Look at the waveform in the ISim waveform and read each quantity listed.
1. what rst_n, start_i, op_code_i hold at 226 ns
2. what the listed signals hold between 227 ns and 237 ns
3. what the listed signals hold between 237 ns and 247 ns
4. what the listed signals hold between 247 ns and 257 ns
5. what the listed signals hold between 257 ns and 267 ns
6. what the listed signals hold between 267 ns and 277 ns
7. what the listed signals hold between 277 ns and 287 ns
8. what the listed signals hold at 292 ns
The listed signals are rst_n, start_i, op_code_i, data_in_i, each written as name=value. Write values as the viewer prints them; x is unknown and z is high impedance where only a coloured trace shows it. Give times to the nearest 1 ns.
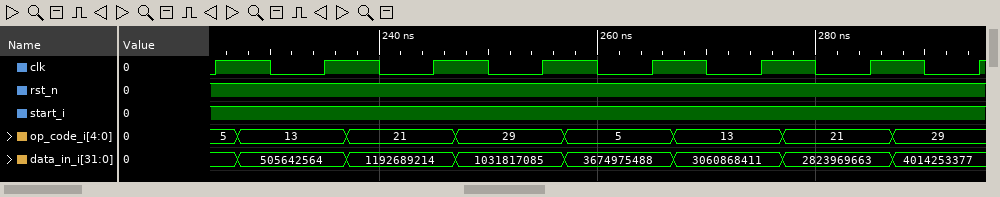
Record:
rst_n=1, start_i=1, op_code_i=5
rst_n=1, start_i=1, op_code_i=13, data_in_i=505642564
rst_n=1, start_i=1, op_code_i=21, data_in_i=1192689214
rst_n=1, start_i=1, op_code_i=29, data_in_i=1031817085
rst_n=1, start_i=1, op_code_i=5, data_in_i=3674975488
rst_n=1, start_i=1, op_code_i=13, data_in_i=3060868411
rst_n=1, start_i=1, op_code_i=21, data_in_i=2823969663
rst_n=1, start_i=1, op_code_i=29, data_in_i=4014253377
